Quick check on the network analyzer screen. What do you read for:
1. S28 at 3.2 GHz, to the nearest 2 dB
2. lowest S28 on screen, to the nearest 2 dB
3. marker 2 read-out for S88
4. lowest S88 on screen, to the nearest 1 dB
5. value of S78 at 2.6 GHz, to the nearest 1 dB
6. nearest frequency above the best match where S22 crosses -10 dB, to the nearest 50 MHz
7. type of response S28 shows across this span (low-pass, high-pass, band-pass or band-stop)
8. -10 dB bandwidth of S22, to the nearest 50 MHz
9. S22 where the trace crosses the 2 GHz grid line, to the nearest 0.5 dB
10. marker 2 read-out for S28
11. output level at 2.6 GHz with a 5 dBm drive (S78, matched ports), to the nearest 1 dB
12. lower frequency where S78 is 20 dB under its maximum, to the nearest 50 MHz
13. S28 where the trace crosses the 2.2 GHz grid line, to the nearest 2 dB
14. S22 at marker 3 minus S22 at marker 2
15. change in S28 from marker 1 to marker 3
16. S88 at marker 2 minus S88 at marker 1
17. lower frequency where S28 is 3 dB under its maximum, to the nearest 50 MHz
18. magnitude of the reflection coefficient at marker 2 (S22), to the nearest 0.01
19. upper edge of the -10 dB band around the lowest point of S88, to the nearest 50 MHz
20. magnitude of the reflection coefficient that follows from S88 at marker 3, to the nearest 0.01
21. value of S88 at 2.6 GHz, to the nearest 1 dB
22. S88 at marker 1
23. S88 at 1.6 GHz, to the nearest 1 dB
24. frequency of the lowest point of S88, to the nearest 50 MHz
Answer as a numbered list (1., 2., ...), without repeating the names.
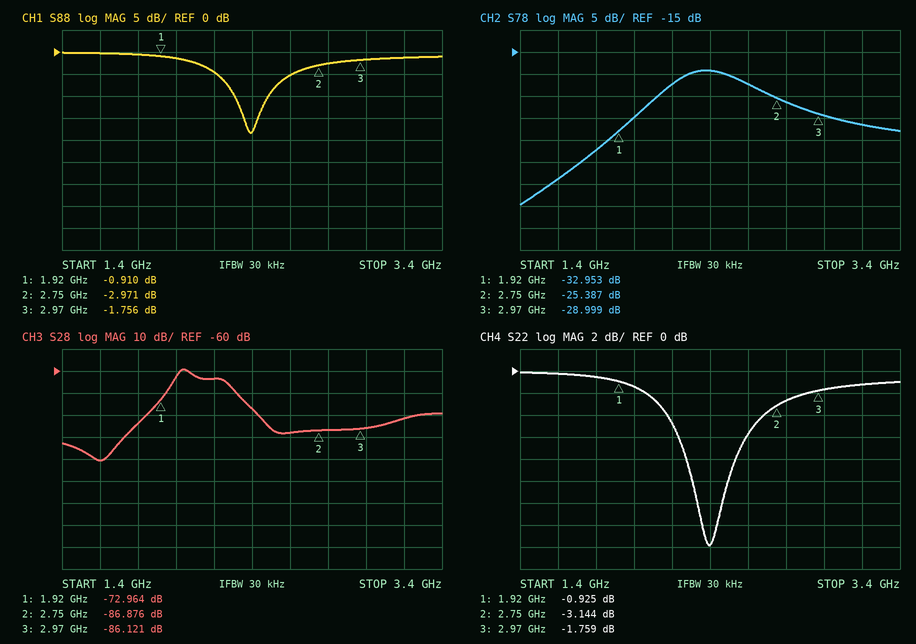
1. -82 dB
2. -100 dB
3. -2.971 dB
4. -18 dB
5. -22 dB
6. 2.50 GHz
7. band-pass
8. 200 MHz
9. -1.5 dB
10. -86.876 dB
11. -17 dBm
12. 1.75 GHz
13. -64 dB
14. 1.385 dB
15. -13.157 dB
16. -2.061 dB
17. 2.00 GHz
18. 0.70
19. 2.50 GHz
20. 0.82
21. -5 dB
22. -0.910 dB
23. 0 dB
24. 2.40 GHz
